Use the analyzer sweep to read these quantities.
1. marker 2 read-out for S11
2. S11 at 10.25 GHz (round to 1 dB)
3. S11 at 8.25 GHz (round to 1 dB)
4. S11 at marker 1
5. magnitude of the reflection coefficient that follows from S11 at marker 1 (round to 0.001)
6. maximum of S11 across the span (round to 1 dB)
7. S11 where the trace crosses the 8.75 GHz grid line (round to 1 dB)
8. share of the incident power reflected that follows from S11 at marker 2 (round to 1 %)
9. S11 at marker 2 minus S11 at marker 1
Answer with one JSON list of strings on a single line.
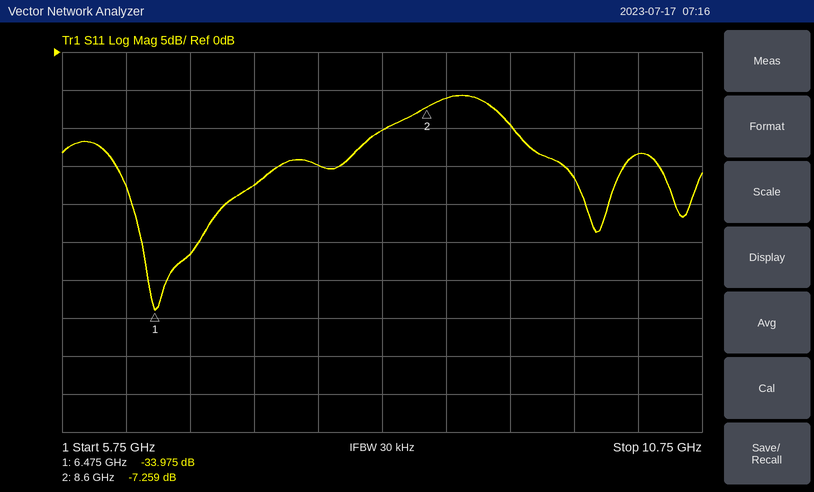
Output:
["-7.259 dB", "-13 dB", "-10 dB", "-33.975 dB", "0.020", "-6 dB", "-6 dB", "19 %", "26.716 dB"]
